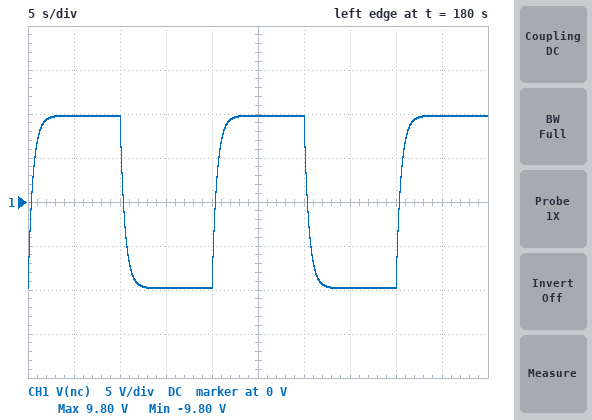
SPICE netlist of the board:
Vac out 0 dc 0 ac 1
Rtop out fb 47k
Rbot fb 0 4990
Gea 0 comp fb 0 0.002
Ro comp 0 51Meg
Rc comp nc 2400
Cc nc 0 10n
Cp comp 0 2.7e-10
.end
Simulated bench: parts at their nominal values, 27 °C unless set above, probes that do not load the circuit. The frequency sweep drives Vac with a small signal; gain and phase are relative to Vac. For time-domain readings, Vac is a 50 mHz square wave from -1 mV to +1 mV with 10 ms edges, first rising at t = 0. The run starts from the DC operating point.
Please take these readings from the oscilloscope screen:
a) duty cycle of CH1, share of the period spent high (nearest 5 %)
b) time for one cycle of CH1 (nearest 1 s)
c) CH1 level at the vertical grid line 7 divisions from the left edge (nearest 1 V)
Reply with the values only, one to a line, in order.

50 %
20 s
-10 V
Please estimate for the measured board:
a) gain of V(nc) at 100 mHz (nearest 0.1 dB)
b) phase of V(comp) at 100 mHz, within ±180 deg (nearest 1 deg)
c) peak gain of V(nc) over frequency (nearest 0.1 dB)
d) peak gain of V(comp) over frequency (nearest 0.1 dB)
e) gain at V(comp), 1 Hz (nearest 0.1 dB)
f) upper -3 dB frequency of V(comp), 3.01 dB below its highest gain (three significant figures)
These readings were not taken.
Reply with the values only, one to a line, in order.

79.4 dB
-18 deg
79.8 dB
79.8 dB
69.1 dB
304 mHz
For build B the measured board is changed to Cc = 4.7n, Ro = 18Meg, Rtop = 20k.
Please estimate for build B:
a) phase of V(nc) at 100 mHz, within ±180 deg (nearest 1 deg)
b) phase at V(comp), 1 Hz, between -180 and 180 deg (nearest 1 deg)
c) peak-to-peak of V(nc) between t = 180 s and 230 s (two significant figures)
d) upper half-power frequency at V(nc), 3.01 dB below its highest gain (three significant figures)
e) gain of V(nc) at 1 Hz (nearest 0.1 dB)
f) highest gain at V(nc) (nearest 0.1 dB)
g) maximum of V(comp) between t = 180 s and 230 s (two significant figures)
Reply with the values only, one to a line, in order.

-3 deg
-29 deg
14 V
1.78 Hz
75.9 dB
77.1 dB
7.2 V
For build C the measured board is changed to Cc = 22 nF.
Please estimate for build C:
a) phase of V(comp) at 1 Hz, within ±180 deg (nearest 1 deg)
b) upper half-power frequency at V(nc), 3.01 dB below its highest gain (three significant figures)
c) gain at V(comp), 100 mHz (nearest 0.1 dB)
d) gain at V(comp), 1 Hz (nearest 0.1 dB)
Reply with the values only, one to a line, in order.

-82 deg
140 mHz
78.0 dB
62.7 dB
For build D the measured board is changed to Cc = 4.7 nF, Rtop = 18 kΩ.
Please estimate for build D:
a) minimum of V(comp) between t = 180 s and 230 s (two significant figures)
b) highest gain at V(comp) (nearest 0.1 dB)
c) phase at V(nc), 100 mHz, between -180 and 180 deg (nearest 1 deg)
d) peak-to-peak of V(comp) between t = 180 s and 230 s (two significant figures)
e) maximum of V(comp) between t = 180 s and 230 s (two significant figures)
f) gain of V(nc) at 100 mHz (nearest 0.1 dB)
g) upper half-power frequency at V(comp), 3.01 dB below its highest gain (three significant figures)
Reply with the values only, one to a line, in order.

-22 V
86.9 dB
-9 deg
44 V
22 V
86.8 dB
628 mHz
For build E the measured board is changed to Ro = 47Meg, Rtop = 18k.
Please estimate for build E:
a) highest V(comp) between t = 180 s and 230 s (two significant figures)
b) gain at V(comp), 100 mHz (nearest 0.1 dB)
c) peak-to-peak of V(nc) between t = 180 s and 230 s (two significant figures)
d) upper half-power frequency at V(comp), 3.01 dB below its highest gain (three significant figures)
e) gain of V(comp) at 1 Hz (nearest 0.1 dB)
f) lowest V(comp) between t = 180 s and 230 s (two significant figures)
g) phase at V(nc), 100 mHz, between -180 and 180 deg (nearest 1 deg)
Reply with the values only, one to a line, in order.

20 V
85.8 dB
41 V
330 mHz
76.1 dB
-20 V
-17 deg
